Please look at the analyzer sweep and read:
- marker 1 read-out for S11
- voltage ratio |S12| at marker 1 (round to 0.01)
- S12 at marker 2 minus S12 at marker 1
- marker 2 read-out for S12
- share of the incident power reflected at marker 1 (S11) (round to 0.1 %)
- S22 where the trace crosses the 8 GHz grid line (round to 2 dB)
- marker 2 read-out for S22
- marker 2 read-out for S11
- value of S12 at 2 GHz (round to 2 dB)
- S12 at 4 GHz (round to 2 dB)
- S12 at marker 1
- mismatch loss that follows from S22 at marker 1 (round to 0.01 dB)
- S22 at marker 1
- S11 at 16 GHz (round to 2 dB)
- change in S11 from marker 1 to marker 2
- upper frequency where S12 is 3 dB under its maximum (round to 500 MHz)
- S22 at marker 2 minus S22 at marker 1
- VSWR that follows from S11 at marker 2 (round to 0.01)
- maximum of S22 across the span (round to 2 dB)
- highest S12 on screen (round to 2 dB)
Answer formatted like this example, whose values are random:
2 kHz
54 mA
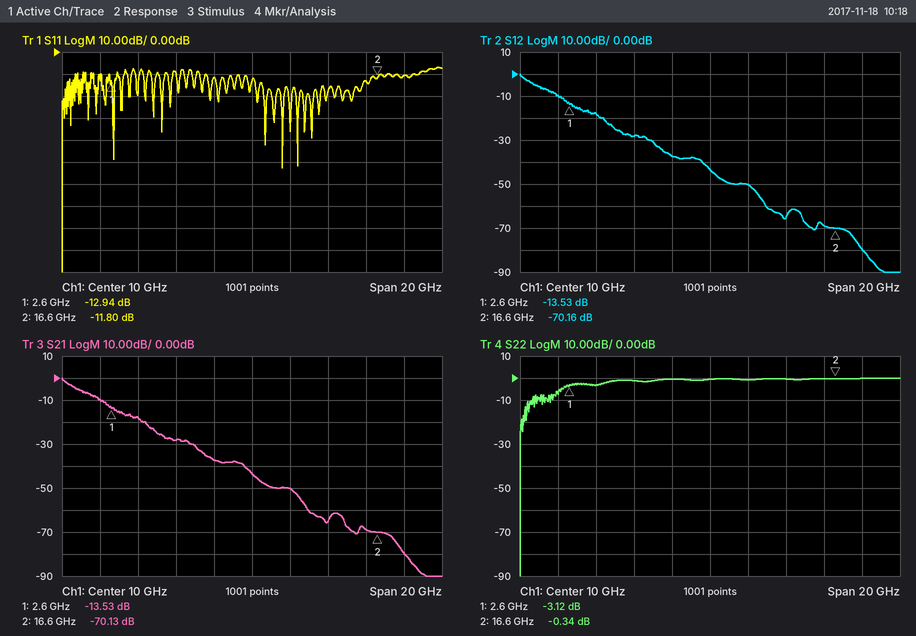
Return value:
-12.94 dB
0.21
-56.63 dB
-70.16 dB
5.1 %
0 dB
-0.34 dB
-11.80 dB
-10 dB
-18 dB
-13.53 dB
2.90 dB
-3.12 dB
-14 dB
1.14 dB
500 MHz
2.78 dB
1.69
0 dB
0 dB
